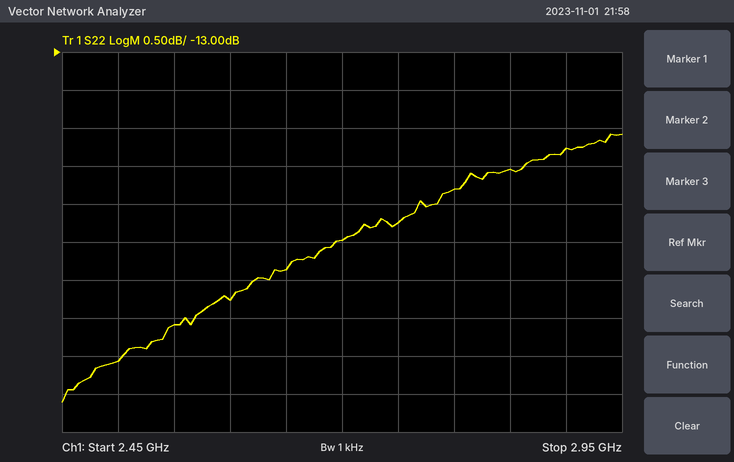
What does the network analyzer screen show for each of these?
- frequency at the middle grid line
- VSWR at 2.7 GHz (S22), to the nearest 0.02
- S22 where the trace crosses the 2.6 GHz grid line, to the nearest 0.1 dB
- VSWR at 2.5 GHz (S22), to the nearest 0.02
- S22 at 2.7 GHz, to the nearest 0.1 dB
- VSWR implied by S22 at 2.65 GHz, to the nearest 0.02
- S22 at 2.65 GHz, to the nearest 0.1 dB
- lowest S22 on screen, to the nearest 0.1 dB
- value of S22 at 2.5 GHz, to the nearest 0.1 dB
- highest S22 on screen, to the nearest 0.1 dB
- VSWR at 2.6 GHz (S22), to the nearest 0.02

2.7 GHz
1.40
-16.3 dB
1.32
-15.5 dB
1.38
-15.9 dB
-17.6 dB
-17.1 dB
-14.1 dB
1.36
